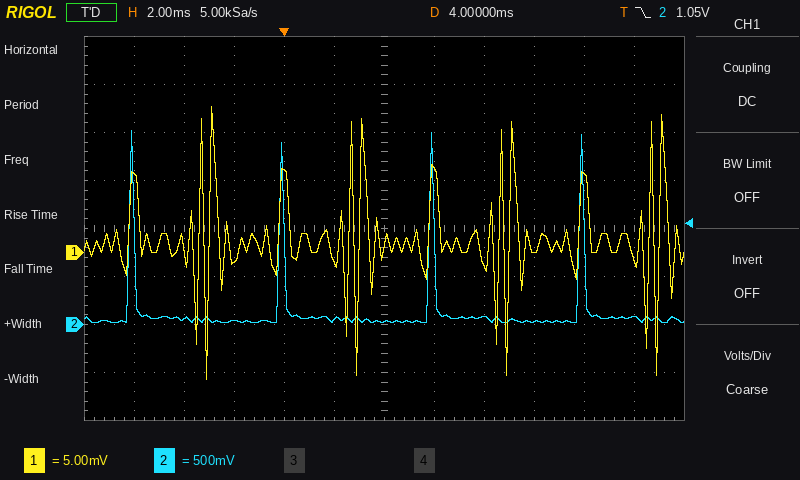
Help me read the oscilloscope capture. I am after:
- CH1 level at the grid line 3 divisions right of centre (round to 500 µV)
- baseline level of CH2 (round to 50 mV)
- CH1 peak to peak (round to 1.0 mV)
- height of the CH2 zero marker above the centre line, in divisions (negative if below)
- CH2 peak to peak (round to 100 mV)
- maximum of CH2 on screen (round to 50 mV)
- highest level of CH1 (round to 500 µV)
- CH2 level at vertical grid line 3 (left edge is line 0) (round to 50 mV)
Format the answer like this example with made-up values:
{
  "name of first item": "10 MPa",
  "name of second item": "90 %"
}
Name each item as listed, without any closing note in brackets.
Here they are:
{
  "CH1 level at the grid line 3 divisions right of centre": "0.0 mV",
  "baseline level of CH2": "50 mV",
  "CH1 peak to peak": "28.0 mV",
  "height of the CH2 zero marker above the centre line, in divisions": "-2.0 div",
  "CH2 peak to peak": "2.00 V",
  "maximum of CH2 on screen": "2.00 V",
  "highest level of CH1": "15.0 mV",
  "CH2 level at vertical grid line 3 (left edge is line 0)": "50 mV"
}
